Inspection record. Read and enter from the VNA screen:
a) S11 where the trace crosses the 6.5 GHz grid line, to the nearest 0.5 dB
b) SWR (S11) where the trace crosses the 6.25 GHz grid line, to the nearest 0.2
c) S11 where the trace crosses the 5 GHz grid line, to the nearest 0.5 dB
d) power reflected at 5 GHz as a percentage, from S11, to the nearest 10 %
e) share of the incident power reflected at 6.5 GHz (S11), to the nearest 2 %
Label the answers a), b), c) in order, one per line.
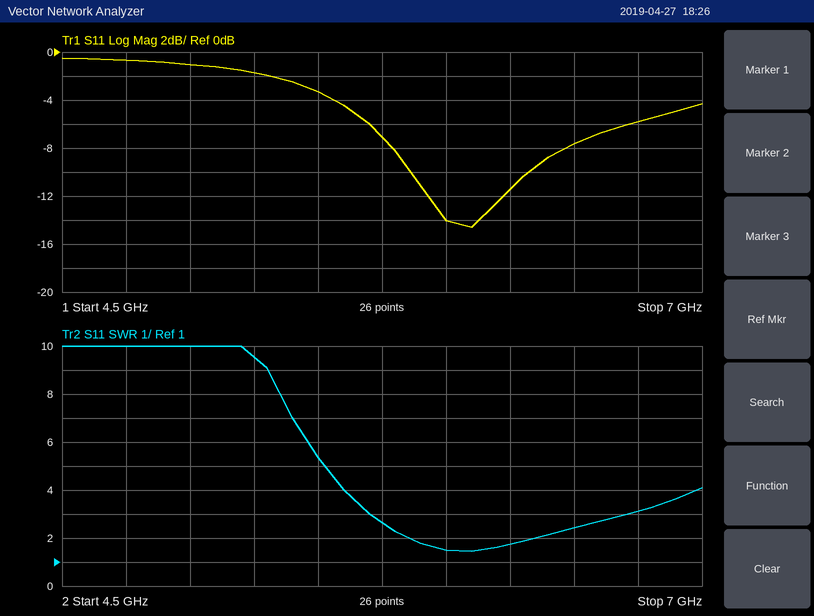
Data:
a) -7.5 dB
b) 1.8
c) -1.0 dB
d) 80 %
e) 18 %
